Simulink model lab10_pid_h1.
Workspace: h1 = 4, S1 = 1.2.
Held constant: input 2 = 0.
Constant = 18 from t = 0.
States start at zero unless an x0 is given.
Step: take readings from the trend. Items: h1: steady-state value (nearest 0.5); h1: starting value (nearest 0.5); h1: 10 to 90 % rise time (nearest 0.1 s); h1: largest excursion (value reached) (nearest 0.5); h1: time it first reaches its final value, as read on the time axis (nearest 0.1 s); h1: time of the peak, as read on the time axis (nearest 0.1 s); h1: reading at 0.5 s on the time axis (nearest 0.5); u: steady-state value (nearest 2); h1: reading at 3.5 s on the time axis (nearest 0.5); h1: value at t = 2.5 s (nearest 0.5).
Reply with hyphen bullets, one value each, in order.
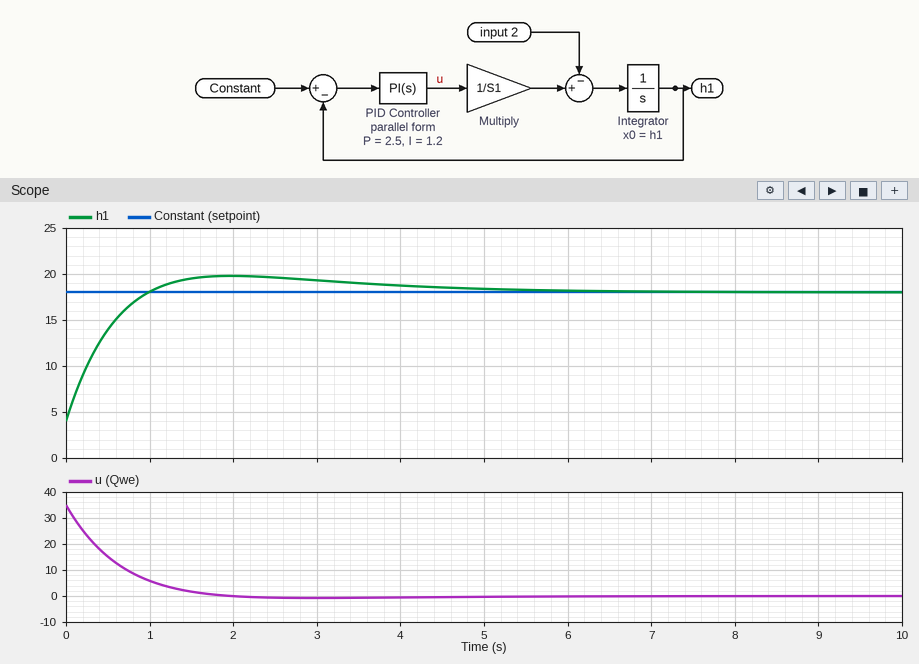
- 18.0
- 4.0
- 0.7 s
- 20.0
- 1.0 s
- 2.0 s
- 14.0
- 0
- 19.0
- 19.5
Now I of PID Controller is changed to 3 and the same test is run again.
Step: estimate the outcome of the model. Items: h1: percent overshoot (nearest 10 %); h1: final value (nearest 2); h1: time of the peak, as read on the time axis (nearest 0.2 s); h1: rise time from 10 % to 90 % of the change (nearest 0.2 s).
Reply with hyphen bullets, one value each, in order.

- 20 %
- 18
- 1.4 s
- 0.6 s
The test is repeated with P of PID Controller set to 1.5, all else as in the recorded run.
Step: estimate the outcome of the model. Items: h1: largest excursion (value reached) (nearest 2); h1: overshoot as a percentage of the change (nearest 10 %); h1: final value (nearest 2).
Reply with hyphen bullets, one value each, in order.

- 22
- 20 %
- 18
